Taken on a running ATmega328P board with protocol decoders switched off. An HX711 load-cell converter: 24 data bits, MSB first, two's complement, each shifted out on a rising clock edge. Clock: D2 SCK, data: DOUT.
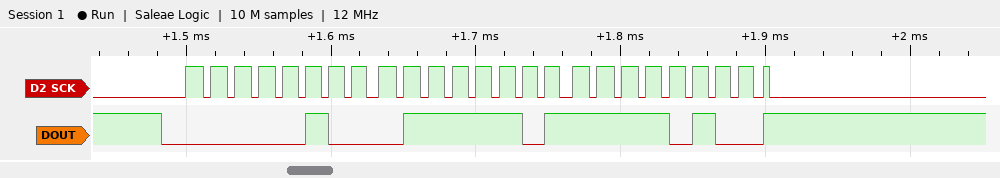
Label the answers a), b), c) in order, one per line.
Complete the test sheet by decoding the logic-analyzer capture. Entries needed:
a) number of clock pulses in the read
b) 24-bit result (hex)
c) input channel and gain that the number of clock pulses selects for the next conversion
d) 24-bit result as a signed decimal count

a) 25
b) 0x047DF4
c) channel A, gain 128
d) 294388
